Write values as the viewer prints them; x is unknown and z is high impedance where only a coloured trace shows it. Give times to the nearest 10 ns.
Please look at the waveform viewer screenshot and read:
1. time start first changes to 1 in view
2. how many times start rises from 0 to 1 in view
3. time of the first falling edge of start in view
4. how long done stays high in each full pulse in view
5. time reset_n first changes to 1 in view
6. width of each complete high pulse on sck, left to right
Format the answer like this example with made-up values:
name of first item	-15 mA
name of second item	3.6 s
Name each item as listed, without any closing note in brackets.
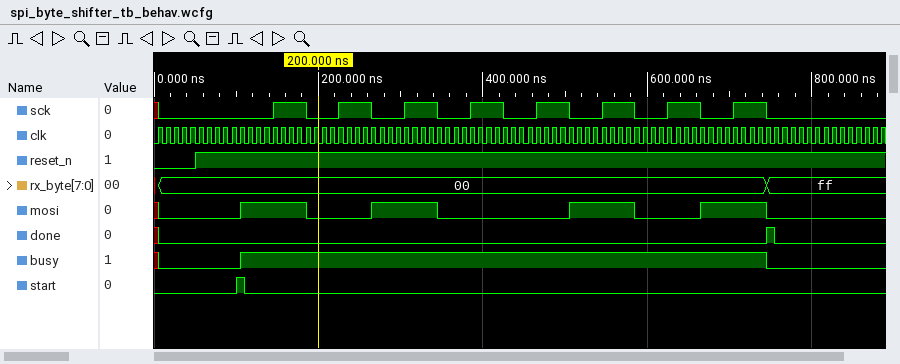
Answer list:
time start first changes to 1 in view	100 ns
how many times start rises from 0 to 1 in view	1
time of the first falling edge of start in view	110 ns
how long done stays high in each full pulse in view	10 ns
time reset_n first changes to 1 in view	50 ns
width of each complete high pulse on sck, left to right	40 ns, 40 ns, 40 ns, 40 ns, 40 ns, 40 ns, 40 ns, 40 ns
